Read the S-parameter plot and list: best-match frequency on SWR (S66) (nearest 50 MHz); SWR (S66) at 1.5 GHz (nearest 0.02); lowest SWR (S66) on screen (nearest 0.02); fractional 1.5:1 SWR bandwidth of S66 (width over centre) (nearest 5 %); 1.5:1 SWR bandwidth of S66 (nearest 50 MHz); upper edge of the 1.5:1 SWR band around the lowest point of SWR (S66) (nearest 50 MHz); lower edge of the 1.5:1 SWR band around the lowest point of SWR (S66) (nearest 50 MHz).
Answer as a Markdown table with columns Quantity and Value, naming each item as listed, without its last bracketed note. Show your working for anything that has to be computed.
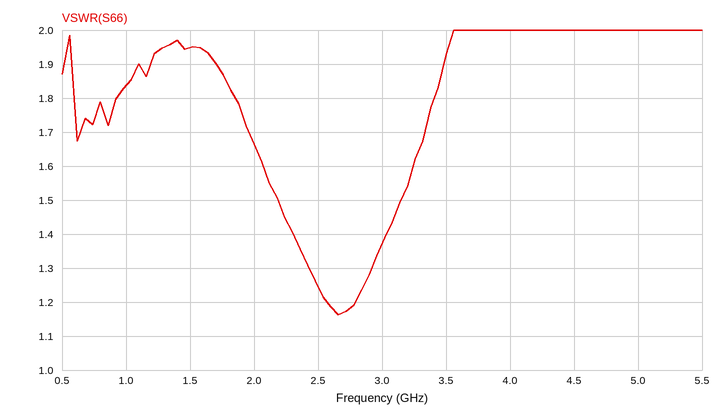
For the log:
| Quantity | Value |
|---|---|
| best-match frequency on SWR (S66) | 2.65 GHz |
| SWR (S66) at 1.5 GHz | 1.94 |
| lowest SWR (S66) on screen | 1.16 |
| fractional 1.5:1 SWR bandwidth of S66 (width over centre) | 950 MHz / 2.675 GHz ≈ 35 % |
| 1.5:1 SWR bandwidth of S66 | 3.15 GHz − 2.20 GHz = 950 MHz |
| upper edge of the 1.5:1 SWR band around the lowest point of SWR (S66) | 3.15 GHz |
| lower edge of the 1.5:1 SWR band around the lowest point of SWR (S66) | 2.20 GHz |
